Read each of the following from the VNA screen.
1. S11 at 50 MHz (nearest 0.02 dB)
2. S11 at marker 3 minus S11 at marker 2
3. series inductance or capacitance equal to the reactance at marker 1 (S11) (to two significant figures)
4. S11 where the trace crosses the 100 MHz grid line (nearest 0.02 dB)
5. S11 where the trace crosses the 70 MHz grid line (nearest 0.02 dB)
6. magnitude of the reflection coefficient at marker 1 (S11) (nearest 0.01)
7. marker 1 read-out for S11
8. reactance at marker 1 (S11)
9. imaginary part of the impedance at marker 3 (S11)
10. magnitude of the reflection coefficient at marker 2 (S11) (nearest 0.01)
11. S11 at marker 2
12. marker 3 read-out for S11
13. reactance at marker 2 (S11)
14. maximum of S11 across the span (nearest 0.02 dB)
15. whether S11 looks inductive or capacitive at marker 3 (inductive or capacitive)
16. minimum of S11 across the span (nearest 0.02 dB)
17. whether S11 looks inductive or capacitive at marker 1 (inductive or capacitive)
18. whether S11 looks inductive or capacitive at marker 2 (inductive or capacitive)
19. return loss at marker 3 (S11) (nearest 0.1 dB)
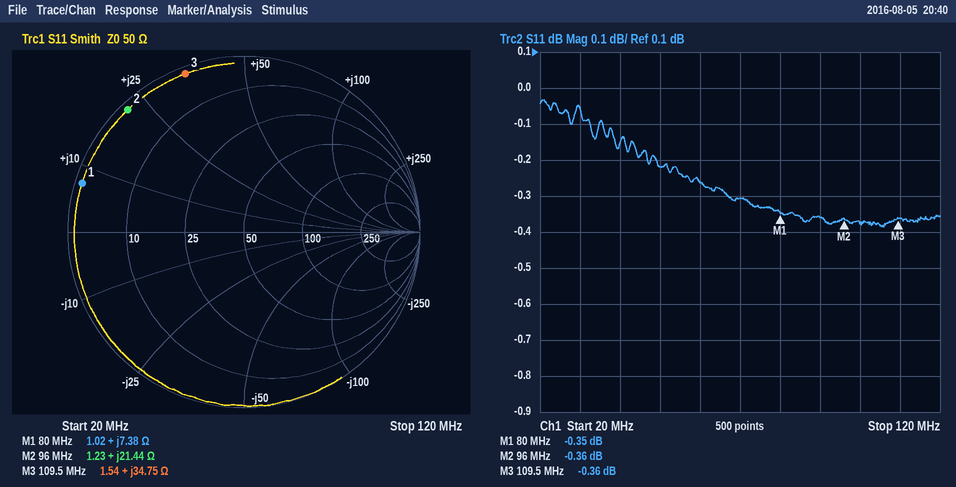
-0.22 dB
0.00 dB
15 nH
-0.38 dB
-0.30 dB
0.96
-0.35 dB
+7.38 Ω
+34.75 Ω
0.96
-0.36 dB
-0.36 dB
+21.44 Ω
-0.04 dB
inductive
-0.38 dB
inductive
inductive
0.4 dB
